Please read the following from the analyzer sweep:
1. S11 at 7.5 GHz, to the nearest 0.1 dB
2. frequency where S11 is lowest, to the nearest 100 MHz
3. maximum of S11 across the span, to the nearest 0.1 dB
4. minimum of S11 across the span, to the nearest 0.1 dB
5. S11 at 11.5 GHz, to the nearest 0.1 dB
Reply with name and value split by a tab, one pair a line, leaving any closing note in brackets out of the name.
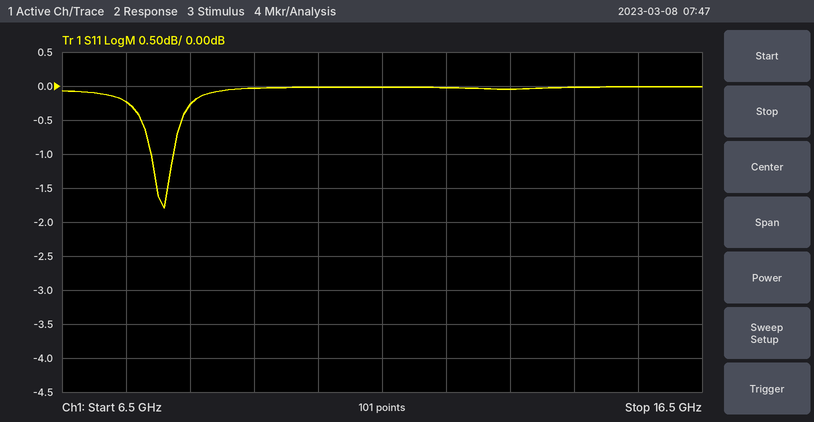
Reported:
S11 at 7.5 GHz, to the nearest 0.1 dB	-0.2 dB
frequency where S11 is lowest, to the nearest 100 MHz	8.1 GHz
maximum of S11 across the span, to the nearest 0.1 dB	0.0 dB
minimum of S11 across the span, to the nearest 0.1 dB	-1.8 dB
S11 at 11.5 GHz, to the nearest 0.1 dB	0.0 dB
